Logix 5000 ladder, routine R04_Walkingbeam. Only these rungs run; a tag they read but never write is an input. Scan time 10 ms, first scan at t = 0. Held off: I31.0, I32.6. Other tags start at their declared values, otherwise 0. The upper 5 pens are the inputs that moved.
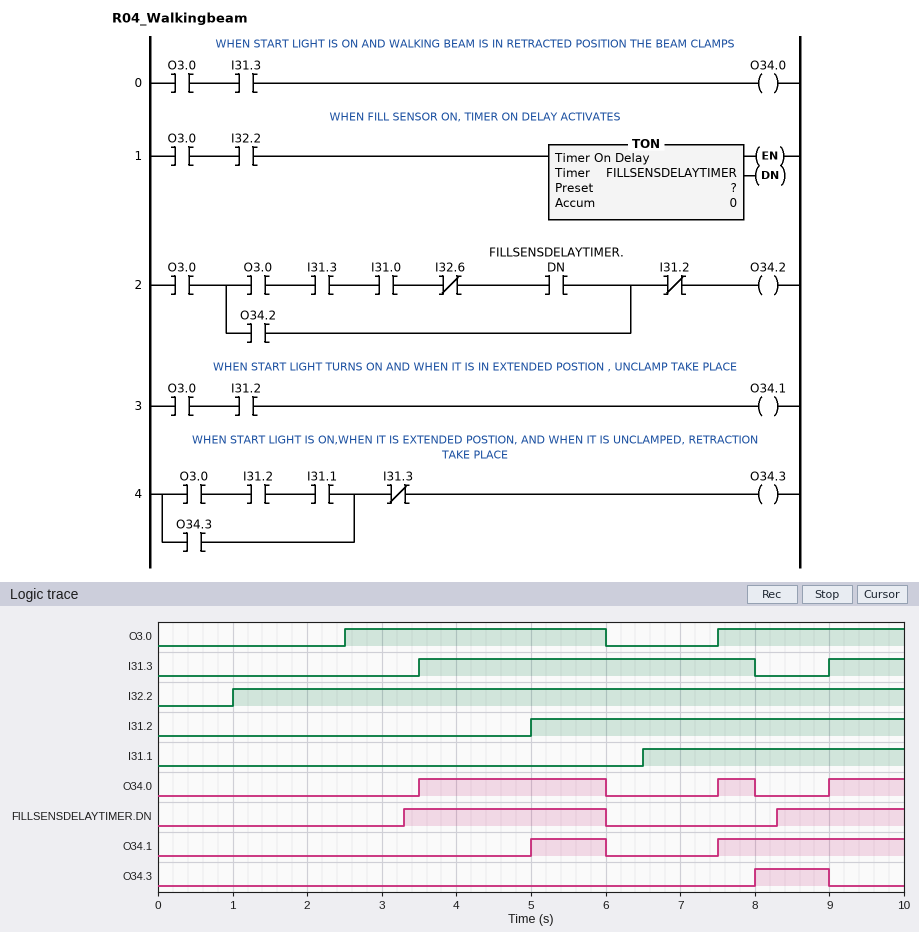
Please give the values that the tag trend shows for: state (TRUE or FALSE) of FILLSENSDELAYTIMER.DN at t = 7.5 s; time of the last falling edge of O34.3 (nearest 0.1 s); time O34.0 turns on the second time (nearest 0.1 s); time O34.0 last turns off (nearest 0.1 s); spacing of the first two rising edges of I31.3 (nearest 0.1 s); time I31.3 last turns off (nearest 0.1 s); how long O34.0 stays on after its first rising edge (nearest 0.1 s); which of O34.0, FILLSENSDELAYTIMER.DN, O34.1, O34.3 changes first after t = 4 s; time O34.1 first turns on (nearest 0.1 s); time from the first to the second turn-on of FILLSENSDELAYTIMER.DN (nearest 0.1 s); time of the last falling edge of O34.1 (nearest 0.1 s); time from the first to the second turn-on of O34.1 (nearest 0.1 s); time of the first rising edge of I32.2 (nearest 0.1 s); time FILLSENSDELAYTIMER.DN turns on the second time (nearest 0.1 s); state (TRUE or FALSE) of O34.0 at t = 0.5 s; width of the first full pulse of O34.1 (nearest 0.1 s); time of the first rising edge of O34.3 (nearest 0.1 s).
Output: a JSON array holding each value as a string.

["FALSE", "9.0 s", "7.5 s", "8.0 s", "5.5 s", "8.0 s", "2.5 s", "O34.1", "5.0 s", "5.0 s", "6.0 s", "2.5 s", "1.0 s", "8.3 s", "FALSE", "1.0 s", "8.0 s"]
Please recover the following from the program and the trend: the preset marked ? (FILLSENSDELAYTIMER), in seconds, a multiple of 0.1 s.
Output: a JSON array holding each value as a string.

["0.8 s"]
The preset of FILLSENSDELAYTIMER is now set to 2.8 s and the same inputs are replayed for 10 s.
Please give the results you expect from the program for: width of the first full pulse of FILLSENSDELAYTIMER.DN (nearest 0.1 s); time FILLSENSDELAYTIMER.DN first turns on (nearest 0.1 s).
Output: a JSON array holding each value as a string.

["0.7 s", "5.3 s"]
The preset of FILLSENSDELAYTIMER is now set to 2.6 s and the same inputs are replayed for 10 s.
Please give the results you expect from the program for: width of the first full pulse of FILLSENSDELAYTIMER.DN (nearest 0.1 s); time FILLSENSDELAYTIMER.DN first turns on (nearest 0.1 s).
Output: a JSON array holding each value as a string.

["0.9 s", "5.1 s"]
